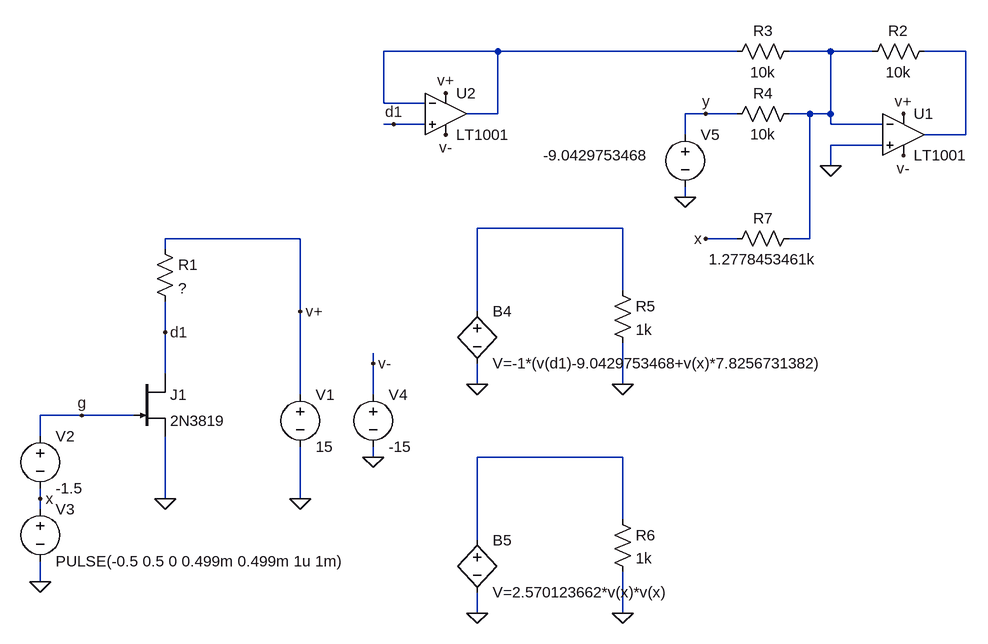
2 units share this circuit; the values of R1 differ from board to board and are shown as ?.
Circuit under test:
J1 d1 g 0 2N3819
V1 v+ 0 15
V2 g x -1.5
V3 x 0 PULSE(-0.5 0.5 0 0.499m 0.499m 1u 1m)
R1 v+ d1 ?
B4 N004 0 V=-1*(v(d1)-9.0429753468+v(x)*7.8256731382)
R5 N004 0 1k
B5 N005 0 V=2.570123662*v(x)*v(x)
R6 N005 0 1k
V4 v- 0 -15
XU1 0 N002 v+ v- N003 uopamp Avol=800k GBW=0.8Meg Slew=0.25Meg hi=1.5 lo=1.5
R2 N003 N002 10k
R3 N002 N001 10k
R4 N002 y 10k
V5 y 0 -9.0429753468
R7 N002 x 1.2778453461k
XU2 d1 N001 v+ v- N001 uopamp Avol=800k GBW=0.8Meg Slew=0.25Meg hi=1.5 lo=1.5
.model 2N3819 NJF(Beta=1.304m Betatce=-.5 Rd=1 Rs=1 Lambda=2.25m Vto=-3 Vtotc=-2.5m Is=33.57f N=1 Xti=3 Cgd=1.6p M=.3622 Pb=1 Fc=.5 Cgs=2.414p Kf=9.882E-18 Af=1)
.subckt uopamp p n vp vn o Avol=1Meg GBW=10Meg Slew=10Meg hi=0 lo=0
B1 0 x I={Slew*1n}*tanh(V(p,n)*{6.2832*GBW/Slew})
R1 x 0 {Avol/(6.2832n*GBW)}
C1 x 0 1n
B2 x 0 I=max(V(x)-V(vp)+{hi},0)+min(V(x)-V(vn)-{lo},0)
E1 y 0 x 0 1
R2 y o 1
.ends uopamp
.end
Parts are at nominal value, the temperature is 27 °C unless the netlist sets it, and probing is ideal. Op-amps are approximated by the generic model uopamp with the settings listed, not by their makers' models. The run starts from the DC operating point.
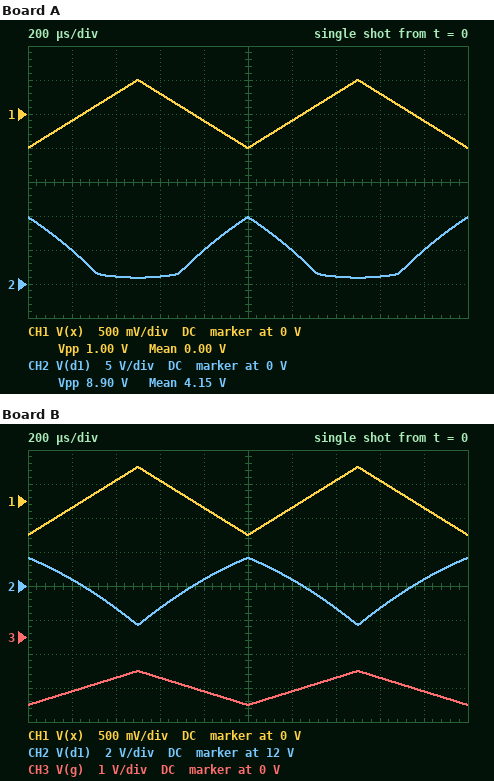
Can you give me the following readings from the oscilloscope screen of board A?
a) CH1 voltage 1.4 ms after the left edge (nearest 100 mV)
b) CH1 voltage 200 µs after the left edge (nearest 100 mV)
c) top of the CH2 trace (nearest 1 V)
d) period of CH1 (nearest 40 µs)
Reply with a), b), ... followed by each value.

a) 300 mV
b) -100 mV
c) 10 V
d) 1.00 ms
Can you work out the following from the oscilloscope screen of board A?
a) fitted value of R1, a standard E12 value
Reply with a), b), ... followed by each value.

a) 3.9 kΩ
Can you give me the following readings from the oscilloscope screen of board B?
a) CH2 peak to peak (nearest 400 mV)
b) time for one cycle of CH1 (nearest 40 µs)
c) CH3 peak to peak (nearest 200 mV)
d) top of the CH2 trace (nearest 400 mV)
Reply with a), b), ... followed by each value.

a) 4.0 V
b) 1.00 ms
c) 1.0 V
d) 13.6 V
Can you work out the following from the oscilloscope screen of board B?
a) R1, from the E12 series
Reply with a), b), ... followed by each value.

a) 1 kΩ
